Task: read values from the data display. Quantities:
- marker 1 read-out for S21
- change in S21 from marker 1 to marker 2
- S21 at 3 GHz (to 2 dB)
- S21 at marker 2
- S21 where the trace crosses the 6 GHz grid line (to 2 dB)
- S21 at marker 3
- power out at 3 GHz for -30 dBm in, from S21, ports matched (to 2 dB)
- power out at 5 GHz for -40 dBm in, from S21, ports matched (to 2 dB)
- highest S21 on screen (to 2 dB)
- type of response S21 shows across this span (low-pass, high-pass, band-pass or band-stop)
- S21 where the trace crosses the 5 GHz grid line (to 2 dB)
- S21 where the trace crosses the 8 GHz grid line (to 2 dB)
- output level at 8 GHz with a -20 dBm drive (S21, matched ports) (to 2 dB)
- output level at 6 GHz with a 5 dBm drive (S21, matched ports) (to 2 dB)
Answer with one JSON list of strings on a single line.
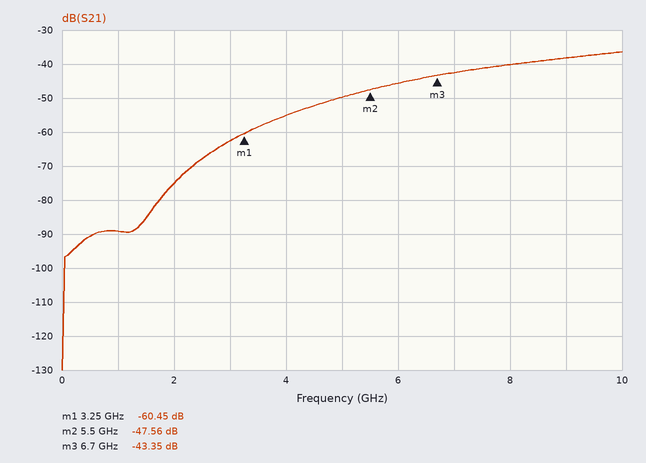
["-60.45 dB", "12.89 dB", "-62 dB", "-47.56 dB", "-46 dB", "-43.35 dB", "-92 dBm", "-90 dBm", "-36 dB", "high-pass", "-50 dB", "-40 dB", "-60 dBm", "-40 dBm"]
